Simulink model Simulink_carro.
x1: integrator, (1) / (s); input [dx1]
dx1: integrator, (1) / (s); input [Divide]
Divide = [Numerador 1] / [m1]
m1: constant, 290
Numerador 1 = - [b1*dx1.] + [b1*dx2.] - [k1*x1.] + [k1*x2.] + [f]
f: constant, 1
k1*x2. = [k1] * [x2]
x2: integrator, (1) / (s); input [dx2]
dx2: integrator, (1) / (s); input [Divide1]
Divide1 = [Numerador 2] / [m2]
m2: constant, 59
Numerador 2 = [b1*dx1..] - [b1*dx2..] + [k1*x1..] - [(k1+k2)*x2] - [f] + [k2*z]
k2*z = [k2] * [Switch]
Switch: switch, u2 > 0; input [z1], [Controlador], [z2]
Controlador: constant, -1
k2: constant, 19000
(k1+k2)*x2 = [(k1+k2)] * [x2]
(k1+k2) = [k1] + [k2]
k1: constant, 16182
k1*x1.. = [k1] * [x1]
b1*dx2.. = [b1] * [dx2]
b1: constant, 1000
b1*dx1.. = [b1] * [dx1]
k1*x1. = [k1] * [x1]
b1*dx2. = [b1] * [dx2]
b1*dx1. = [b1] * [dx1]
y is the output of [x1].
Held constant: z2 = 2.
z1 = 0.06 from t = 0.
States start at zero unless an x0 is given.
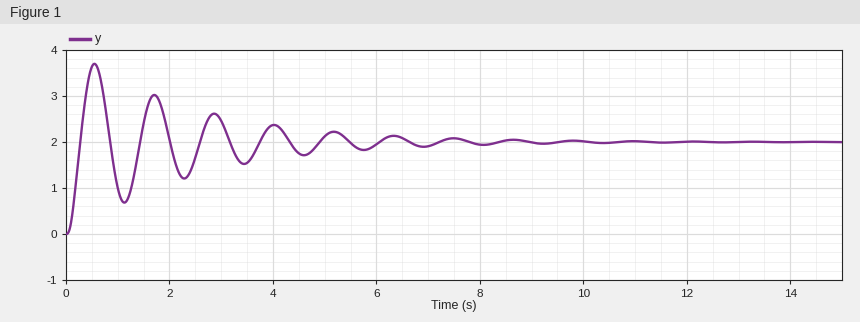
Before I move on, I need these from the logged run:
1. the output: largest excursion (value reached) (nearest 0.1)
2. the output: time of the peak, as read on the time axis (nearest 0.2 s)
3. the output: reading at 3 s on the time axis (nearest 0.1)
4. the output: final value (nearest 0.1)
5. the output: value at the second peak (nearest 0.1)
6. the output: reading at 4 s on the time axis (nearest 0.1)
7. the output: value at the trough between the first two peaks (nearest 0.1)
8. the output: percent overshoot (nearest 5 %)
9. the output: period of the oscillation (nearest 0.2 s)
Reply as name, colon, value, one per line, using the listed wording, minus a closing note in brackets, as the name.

the output: largest excursion (value reached): 3.7
the output: time of the peak, as read on the time axis: 0.6 s
the output: reading at 3 s on the time axis: 2.5
the output: final value: 2.0
the output: value at the second peak: 3.0
the output: reading at 4 s on the time axis: 2.4
the output: value at the trough between the first two peaks: 0.7
the output: percent overshoot: 85 %
the output: period of the oscillation: 1.2 s
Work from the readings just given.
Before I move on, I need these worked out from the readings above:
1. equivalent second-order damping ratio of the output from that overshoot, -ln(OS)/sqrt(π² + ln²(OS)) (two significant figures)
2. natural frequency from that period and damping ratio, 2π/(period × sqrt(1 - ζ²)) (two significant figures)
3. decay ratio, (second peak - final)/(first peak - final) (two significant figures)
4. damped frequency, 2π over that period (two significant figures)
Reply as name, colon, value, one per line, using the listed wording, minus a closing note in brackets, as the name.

equivalent second-order damping ratio of the output from that overshoot, -ln(OS)/sqrt(π² + ln²(OS)): 0.052
natural frequency from that period and damping ratio, 2π/(period × sqrt(1 - ζ²)): 5.2 rad/s
decay ratio, (second peak - final)/(first peak - final): 0.59
damped frequency, 2π over that period: 5.2 rad/s
